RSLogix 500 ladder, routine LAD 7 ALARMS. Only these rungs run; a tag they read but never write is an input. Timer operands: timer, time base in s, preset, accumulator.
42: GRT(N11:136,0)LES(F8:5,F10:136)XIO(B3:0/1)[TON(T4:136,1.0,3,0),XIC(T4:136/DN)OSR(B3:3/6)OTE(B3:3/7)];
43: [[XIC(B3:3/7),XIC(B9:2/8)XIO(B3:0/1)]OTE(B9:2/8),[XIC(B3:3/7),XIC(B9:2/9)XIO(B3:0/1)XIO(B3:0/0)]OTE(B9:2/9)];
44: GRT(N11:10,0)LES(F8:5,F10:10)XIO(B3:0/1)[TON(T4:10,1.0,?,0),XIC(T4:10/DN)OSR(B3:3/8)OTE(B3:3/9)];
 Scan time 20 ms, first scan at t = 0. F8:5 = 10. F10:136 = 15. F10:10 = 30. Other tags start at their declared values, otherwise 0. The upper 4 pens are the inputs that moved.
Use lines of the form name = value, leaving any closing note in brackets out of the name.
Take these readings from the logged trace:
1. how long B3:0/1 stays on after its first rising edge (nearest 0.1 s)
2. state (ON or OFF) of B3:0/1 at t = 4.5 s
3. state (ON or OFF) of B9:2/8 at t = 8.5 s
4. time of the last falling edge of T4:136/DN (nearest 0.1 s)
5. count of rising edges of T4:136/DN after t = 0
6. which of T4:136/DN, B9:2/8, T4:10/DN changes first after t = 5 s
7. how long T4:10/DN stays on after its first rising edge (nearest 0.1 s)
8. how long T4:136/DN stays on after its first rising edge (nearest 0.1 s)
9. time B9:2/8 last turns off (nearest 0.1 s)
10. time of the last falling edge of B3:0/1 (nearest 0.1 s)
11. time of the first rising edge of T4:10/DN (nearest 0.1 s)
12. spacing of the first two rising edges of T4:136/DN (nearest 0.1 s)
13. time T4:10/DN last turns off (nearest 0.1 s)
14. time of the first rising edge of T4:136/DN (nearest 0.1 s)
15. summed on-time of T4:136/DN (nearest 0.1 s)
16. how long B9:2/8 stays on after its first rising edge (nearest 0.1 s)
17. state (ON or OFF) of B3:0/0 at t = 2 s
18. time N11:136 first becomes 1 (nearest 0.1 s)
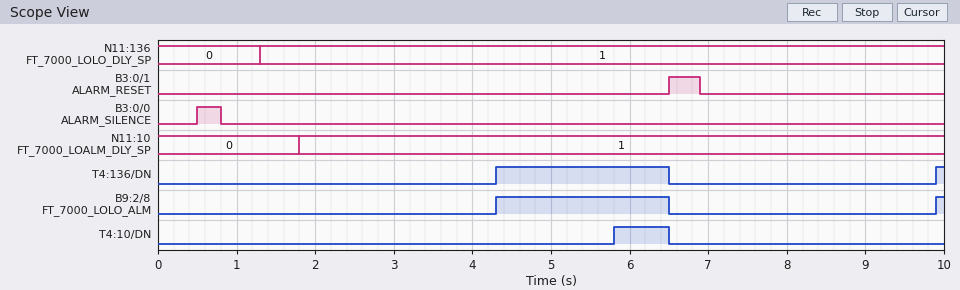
how long B3:0/1 stays on after its first rising edge = 0.4 s
state (ON or OFF) of B3:0/1 at t = 4.5 s = OFF
state (ON or OFF) of B9:2/8 at t = 8.5 s = OFF
time of the last falling edge of T4:136/DN = 6.5 s
count of rising edges of T4:136/DN after t = 0 = 2
which of T4:136/DN, B9:2/8, T4:10/DN changes first after t = 5 s = T4:10/DN
how long T4:10/DN stays on after its first rising edge = 0.7 s
how long T4:136/DN stays on after its first rising edge = 2.2 s
time B9:2/8 last turns off = 6.5 s
time of the last falling edge of B3:0/1 = 6.9 s
time of the first rising edge of T4:10/DN = 5.8 s
spacing of the first two rising edges of T4:136/DN = 5.6 s
time T4:10/DN last turns off = 6.5 s
time of the first rising edge of T4:136/DN = 4.3 s
summed on-time of T4:136/DN = 2.3 s
how long B9:2/8 stays on after its first rising edge = 2.2 s
state (ON or OFF) of B3:0/0 at t = 2 s = OFF
time N11:136 first becomes 1 = 1.3 s
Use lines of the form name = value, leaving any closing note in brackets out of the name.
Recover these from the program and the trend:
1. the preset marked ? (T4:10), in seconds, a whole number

the preset marked ? (T4:10), in seconds, a whole number = 4 s
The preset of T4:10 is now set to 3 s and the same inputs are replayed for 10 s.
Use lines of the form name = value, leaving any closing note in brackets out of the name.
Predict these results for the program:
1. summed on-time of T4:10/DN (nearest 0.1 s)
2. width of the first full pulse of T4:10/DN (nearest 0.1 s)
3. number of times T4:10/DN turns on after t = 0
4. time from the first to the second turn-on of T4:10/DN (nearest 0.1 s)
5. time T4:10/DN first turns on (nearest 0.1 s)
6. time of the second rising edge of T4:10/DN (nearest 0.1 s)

summed on-time of T4:10/DN = 1.8 s
width of the first full pulse of T4:10/DN = 1.7 s
number of times T4:10/DN turns on after t = 0 = 2
time from the first to the second turn-on of T4:10/DN = 5.1 s
time T4:10/DN first turns on = 4.8 s
time of the second rising edge of T4:10/DN = 9.9 s
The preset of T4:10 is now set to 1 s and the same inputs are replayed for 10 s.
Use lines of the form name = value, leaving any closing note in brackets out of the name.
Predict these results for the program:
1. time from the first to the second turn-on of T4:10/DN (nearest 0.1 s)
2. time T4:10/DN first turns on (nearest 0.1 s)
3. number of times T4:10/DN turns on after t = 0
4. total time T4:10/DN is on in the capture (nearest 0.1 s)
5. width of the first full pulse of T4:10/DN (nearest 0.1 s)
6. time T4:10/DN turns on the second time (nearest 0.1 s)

time from the first to the second turn-on of T4:10/DN = 5.1 s
time T4:10/DN first turns on = 2.8 s
number of times T4:10/DN turns on after t = 0 = 2
total time T4:10/DN is on in the capture = 5.8 s
width of the first full pulse of T4:10/DN = 3.7 s
time T4:10/DN turns on the second time = 7.9 s
